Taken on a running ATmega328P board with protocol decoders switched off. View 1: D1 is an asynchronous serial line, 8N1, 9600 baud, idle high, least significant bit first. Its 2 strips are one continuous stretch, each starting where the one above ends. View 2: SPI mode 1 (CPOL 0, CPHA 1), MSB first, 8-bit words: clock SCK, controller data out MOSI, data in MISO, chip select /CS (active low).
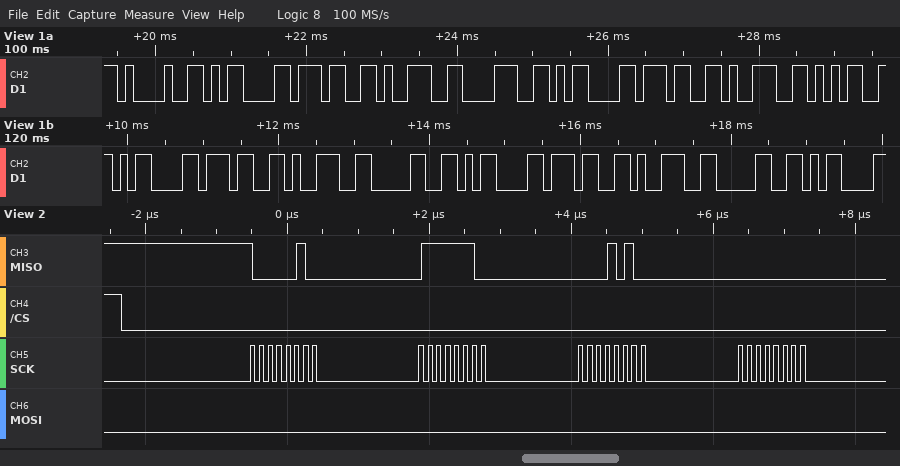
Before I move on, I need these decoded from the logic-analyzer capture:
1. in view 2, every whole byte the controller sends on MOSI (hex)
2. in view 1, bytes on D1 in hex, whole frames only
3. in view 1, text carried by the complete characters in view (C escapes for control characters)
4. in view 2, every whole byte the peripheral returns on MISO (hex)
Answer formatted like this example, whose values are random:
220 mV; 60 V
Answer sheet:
00 00 00 00; 0x21 0x0D 0x37 0x39 0x38 0x0D 0x37 0x39 0x35 0x0D 0x37 0x39 0x30 0x0D 0x37 0x39 0x30 0x0D; "!\r798\r795\r790\r790\r"; 04 FC 14 00
